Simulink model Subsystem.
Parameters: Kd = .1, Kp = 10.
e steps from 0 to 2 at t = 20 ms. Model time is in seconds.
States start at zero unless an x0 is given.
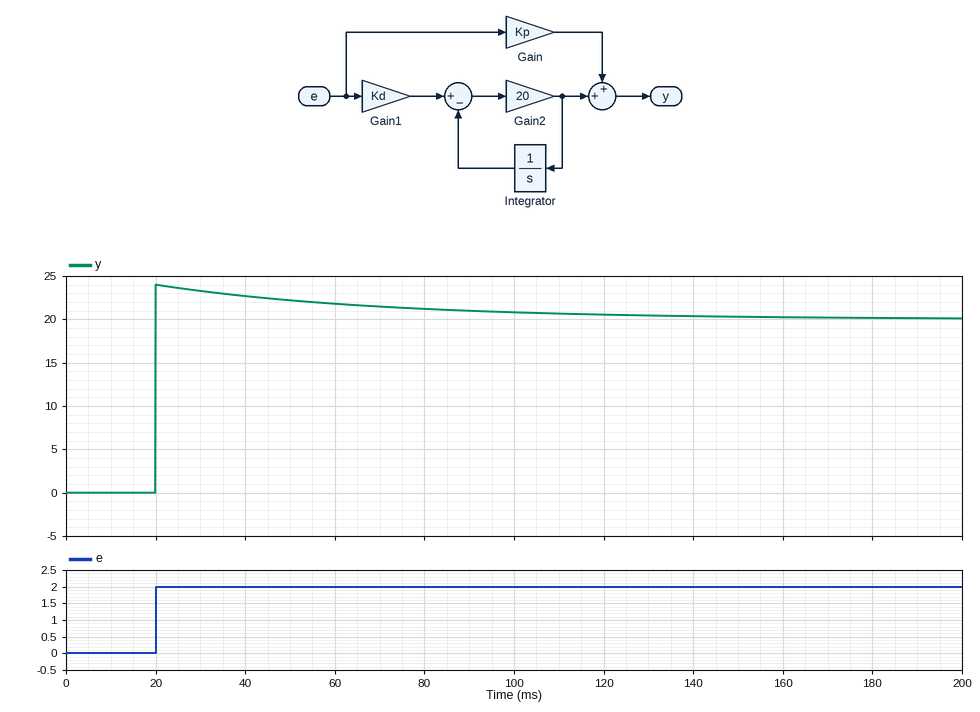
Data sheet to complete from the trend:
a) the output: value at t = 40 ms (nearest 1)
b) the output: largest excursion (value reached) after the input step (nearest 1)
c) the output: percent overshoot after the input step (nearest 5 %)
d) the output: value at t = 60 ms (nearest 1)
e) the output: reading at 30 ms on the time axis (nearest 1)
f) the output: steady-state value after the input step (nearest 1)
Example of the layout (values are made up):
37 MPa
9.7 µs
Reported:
23
24
20 %
22
23
20
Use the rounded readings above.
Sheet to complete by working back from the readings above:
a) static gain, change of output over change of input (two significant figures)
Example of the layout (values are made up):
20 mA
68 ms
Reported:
10
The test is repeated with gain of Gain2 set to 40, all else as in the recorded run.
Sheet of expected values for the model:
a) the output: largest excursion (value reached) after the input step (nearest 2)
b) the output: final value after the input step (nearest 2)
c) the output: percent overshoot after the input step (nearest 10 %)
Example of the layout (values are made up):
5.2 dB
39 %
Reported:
28
20
40 %
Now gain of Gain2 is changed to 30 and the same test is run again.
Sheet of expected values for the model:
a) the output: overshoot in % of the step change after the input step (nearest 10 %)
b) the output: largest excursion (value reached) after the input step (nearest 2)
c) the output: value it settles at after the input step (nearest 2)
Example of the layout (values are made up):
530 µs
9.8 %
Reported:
30 %
26
20
